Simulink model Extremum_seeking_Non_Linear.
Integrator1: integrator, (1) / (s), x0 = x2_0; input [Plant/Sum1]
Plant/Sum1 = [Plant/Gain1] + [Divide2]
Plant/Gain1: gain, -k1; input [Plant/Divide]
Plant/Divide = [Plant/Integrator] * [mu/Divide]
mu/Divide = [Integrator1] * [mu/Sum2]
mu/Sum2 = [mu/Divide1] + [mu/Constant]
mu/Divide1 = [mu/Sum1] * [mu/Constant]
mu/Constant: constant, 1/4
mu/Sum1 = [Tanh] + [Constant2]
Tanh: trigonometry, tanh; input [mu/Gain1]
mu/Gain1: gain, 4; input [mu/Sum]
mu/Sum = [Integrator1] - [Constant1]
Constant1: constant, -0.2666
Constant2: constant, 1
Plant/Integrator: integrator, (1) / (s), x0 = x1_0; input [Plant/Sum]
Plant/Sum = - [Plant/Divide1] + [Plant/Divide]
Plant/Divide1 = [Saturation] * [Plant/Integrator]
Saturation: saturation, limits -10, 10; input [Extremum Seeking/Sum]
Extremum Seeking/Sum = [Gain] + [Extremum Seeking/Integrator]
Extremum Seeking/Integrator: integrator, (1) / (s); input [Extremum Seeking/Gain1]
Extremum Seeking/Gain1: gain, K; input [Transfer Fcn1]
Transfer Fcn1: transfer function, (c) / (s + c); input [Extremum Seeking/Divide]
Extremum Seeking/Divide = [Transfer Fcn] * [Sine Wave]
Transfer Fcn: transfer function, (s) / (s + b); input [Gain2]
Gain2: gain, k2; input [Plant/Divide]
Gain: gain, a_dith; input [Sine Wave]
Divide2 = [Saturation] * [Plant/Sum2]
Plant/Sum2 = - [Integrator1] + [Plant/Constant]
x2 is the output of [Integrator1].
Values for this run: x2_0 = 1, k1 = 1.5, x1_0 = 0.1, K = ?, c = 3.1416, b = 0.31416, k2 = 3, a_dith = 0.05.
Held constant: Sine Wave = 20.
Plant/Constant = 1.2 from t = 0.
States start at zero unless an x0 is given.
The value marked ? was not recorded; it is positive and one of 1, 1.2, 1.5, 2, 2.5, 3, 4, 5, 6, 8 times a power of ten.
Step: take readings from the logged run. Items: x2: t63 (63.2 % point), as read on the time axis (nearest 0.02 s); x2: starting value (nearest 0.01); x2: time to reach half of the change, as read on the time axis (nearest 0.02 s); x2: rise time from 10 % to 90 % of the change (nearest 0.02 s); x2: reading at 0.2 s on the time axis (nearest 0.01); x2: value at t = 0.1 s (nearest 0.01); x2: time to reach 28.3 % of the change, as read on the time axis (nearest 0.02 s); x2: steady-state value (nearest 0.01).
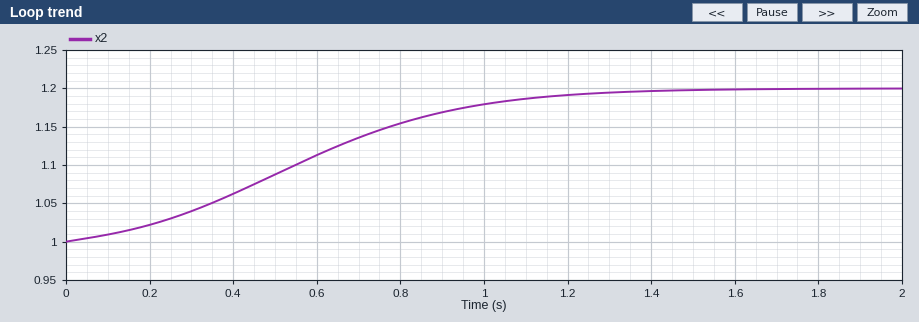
0.66 s
1.00
0.54 s
0.82 s
1.02
1.01
0.38 s
1.20
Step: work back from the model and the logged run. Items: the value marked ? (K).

2
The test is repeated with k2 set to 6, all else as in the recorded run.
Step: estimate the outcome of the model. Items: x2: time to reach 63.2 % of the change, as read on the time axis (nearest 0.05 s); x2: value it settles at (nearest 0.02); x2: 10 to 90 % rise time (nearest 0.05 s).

0.50 s
1.20
0.60 s
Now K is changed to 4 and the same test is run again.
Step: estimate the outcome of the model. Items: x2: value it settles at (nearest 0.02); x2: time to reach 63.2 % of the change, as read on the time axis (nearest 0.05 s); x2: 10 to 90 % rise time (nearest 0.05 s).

1.20
0.50 s
0.60 s
